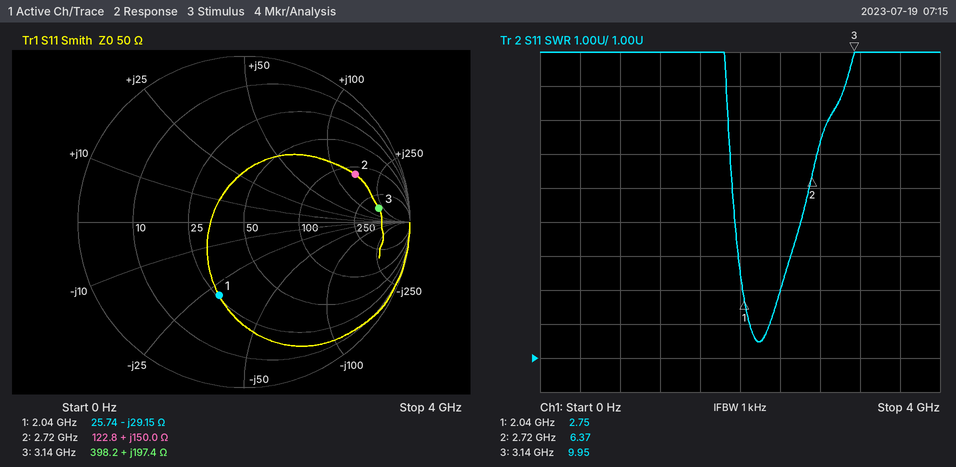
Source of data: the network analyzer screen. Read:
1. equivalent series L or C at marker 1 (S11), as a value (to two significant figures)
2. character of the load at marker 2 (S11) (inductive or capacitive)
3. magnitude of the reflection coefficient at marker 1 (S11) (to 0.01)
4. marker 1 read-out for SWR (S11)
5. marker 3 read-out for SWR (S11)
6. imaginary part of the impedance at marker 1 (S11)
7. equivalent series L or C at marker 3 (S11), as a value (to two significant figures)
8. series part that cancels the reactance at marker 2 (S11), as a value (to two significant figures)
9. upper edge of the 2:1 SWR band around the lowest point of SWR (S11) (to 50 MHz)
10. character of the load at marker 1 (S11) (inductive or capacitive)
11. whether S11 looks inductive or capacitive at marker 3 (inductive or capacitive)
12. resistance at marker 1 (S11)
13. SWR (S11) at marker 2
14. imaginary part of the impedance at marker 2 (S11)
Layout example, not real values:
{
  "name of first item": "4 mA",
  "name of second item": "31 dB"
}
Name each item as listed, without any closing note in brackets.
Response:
{
  "equivalent series L or C at marker 1 (S11), as a value": "2.7 pF",
  "character of the load at marker 2 (S11)": "inductive",
  "magnitude of the reflection coefficient at marker 1 (S11)": "0.47",
  "marker 1 read-out for SWR": "2.75",
  "marker 3 read-out for SWR": "9.95",
  "imaginary part of the impedance at marker 1": "-29.15 Ω",
  "equivalent series L or C at marker 3 (S11), as a value": "10 nH",
  "series part that cancels the reactance at marker 2 (S11), as a value": "390 fF",
  "upper edge of the 2:1 SWR band around the lowest point of SWR (S11)": "2.30 GHz",
  "character of the load at marker 1 (S11)": "capacitive",
  "whether S11 looks inductive or capacitive at marker 3": "inductive",
  "resistance at marker 1": "25.74 Ω",
  "SWR (S11) at marker 2": "6.37",
  "imaginary part of the impedance at marker 2": "+150.0 Ω"
}
